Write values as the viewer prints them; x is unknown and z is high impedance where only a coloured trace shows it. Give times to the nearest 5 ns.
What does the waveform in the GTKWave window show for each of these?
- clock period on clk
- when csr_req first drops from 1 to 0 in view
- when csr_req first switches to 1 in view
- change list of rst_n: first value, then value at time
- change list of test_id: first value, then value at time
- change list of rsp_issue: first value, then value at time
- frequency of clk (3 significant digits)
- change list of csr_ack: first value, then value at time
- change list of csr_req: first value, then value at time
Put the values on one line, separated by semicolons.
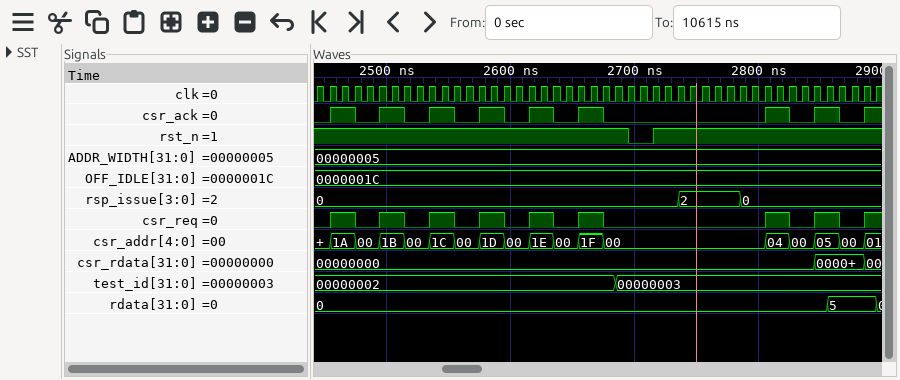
10 ns; 2475 ns; 2455 ns; 1, 0 at 2695 ns, 1 at 2715 ns; 00000002, 00000003 at 2685 ns; 0, 2 at 2735 ns, 0 at 2785 ns; 100 MHz; 0, 1 at 2455 ns, 0 at 2475 ns, 1 at 2495 ns, 0 at 2515 ns, 1 at 2535 ns, 0 at 2555 ns, 1 at 2575 ns, 0 at 2595 ns, 1 at 2615 ns, 0 at 2635 ns, 1 at 2655 ns, 0 at 2675 ns, 1 at 2805 ns, 0 at 2825 ns, 1 at 2845 ns, 0 at 2865 ns, 1 at 2885 ns; 0, 1 at 2455 ns, 0 at 2475 ns, 1 at 2495 ns, 0 at 2515 ns, 1 at 2535 ns, 0 at 2555 ns, 1 at 2575 ns, 0 at 2595 ns, 1 at 2615 ns, 0 at 2635 ns, 1 at 2655 ns, 0 at 2675 ns, 1 at 2805 ns, 0 at 2825 ns, 1 at 2845 ns, 0 at 2865 ns, 1 at 2885 ns
